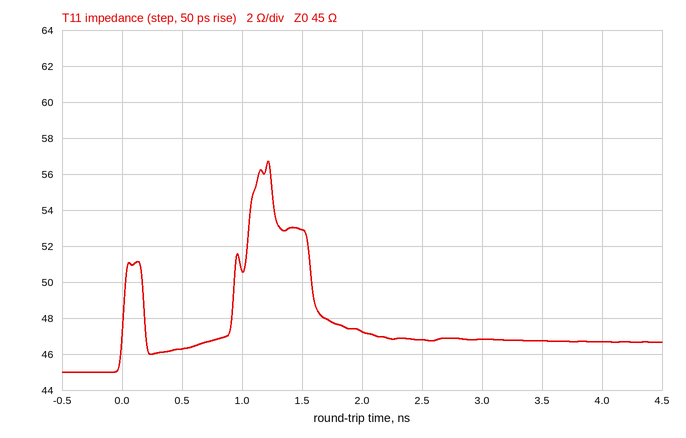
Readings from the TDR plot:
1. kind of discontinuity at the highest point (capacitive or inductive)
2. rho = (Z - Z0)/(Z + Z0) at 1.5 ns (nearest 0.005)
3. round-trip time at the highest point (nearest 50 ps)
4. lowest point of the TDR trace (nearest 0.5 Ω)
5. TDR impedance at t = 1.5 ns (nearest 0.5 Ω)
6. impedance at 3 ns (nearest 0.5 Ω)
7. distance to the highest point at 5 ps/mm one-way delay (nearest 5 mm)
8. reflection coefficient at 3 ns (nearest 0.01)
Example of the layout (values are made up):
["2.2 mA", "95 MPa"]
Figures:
["inductive", "+0.080", "1.20 ns", "45.0 Ω", "53.0 Ω", "47.0 Ω", "120 mm", "+0.02"]
